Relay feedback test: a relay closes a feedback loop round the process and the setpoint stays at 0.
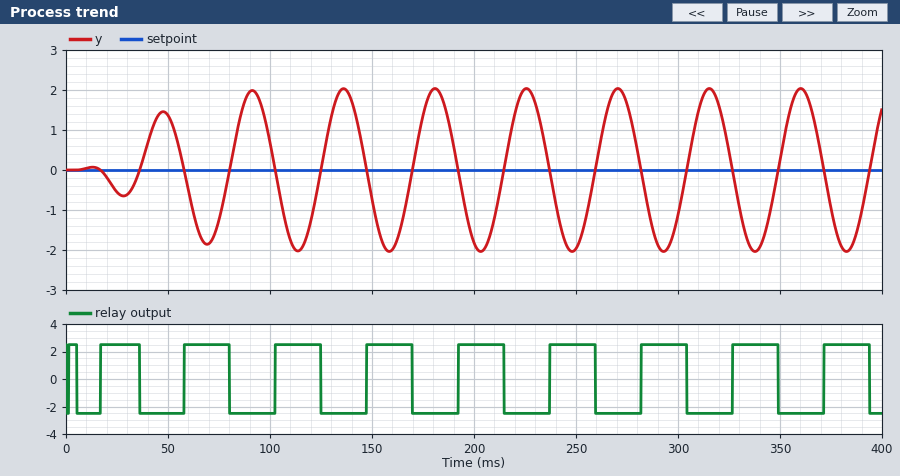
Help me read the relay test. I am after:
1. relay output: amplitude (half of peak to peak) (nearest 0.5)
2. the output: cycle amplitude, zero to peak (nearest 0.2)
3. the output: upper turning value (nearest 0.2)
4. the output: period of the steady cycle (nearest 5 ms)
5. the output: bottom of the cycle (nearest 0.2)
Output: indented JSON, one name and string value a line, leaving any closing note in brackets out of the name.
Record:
{
  "relay output: amplitude (half of peak to peak)": "2.5",
  "the output: cycle amplitude, zero to peak": "2.0",
  "the output: upper turning value": "2.0",
  "the output: period of the steady cycle": "45 ms",
  "the output: bottom of the cycle": "-2.0"
}
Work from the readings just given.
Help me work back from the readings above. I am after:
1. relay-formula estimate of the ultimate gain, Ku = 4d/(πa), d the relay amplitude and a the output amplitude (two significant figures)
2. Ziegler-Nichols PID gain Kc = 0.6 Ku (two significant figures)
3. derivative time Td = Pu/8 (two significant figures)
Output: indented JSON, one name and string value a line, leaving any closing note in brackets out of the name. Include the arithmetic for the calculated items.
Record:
{
  "relay-formula estimate of the ultimate gain, Ku = 4d/(πa), d the relay amplitude and a the output amplitude": "4 × 2.5 / (π × 2) = 1.6",
  "Ziegler-Nichols PID gain Kc = 0.6 Ku": "0.6 × 1.6 = 0.96",
  "derivative time Td = Pu/8": "45 / 8 = 5.6 ms"
}
